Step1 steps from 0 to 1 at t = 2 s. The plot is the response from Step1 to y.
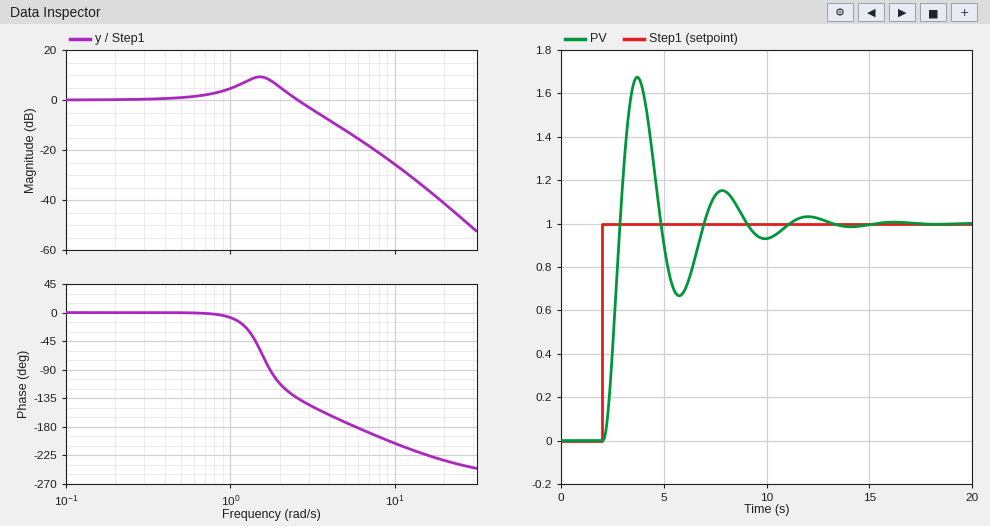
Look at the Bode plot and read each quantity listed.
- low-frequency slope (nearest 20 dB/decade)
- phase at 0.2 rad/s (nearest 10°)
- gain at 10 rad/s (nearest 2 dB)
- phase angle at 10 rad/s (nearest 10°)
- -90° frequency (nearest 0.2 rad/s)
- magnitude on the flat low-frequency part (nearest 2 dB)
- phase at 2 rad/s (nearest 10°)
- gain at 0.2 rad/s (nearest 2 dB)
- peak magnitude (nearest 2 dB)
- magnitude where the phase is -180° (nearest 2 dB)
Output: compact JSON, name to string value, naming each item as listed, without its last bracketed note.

{"low-frequency slope": "0 dB/decade", "phase at 0.2 rad/s": "0°", "gain at 10 rad/s": "-26 dB", "phase angle at 10 rad/s": "-210°", "-90° frequency": "1.8 rad/s", "magnitude on the flat low-frequency part": "0 dB", "phase at 2 rad/s": "-110°", "gain at 0.2 rad/s": "0 dB", "peak magnitude": "10 dB", "magnitude where the phase is -180°": "-14 dB"}
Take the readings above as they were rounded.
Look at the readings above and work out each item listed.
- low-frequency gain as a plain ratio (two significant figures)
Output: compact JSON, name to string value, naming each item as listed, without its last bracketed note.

{"low-frequency gain as a plain ratio": "1.0"}
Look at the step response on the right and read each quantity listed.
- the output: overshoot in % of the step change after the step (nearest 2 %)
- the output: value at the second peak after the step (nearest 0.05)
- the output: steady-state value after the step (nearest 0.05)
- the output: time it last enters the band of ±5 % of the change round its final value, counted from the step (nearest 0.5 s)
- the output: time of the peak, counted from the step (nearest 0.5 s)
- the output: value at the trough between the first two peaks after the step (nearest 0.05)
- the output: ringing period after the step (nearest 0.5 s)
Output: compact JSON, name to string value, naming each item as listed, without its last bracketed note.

{"the output: overshoot in % of the step change after the step": "68 %", "the output: value at the second peak after the step": "1.15", "the output: steady-state value after the step": "1.00", "the output: time it last enters the band of ±5 % of the change round its final value, counted from the step": "8.5 s", "the output: time of the peak, counted from the step": "1.5 s", "the output: value at the trough between the first two peaks after the step": "0.65", "the output: ringing period after the step": "4.0 s"}
